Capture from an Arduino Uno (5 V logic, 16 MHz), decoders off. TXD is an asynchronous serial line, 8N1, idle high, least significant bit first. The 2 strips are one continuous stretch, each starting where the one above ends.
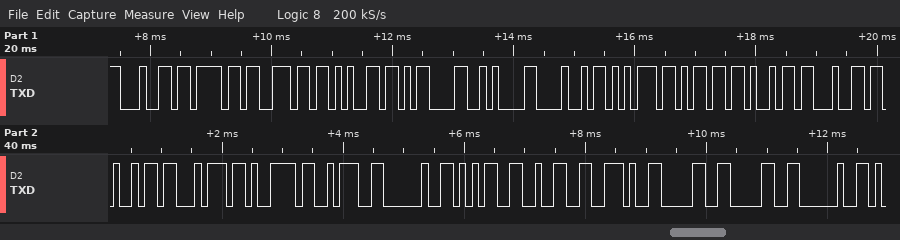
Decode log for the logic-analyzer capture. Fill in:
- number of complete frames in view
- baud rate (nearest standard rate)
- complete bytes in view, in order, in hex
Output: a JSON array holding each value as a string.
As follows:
["22", "9600 baud", "0x64 0x6F 0x6E 0x65 0x0D 0x0A 0x48 0x75 0x6D 0x69 0x64 0x69 0x74 0x79 0x3A 0x20 0x35 0x32 0x2E 0x30 0x30 0x20"]
